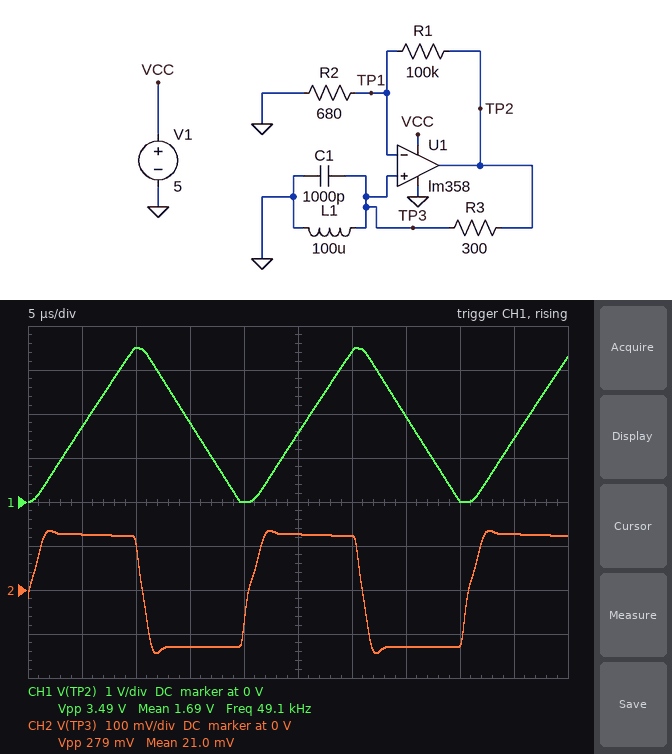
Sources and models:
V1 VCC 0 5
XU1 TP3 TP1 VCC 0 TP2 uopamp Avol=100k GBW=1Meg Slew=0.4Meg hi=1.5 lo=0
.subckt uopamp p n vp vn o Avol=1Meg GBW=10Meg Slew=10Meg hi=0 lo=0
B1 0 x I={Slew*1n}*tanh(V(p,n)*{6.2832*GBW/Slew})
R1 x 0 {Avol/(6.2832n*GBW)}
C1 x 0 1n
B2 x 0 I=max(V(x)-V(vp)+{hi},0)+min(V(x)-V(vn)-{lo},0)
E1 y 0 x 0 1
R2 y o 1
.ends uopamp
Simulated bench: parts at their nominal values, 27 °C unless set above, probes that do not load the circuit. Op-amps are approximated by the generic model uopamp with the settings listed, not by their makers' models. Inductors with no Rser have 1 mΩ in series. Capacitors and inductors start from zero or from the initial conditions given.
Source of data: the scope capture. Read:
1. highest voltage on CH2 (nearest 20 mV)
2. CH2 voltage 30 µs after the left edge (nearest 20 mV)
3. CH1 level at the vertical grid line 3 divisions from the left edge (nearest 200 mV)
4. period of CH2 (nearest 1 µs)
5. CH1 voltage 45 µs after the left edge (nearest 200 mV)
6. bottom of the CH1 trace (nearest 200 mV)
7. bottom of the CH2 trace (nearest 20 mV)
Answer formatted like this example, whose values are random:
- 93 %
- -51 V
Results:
- 140 mV
- 120 mV
- 1.8 V
- 20 µs
- 1.4 V
- 0 V
- -140 mV
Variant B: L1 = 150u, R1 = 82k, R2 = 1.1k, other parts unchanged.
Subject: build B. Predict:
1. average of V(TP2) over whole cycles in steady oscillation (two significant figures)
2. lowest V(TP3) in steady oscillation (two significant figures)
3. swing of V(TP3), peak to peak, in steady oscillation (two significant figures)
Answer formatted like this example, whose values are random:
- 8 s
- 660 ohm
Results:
- 1.7 V
- -210 mV
- 420 mV
